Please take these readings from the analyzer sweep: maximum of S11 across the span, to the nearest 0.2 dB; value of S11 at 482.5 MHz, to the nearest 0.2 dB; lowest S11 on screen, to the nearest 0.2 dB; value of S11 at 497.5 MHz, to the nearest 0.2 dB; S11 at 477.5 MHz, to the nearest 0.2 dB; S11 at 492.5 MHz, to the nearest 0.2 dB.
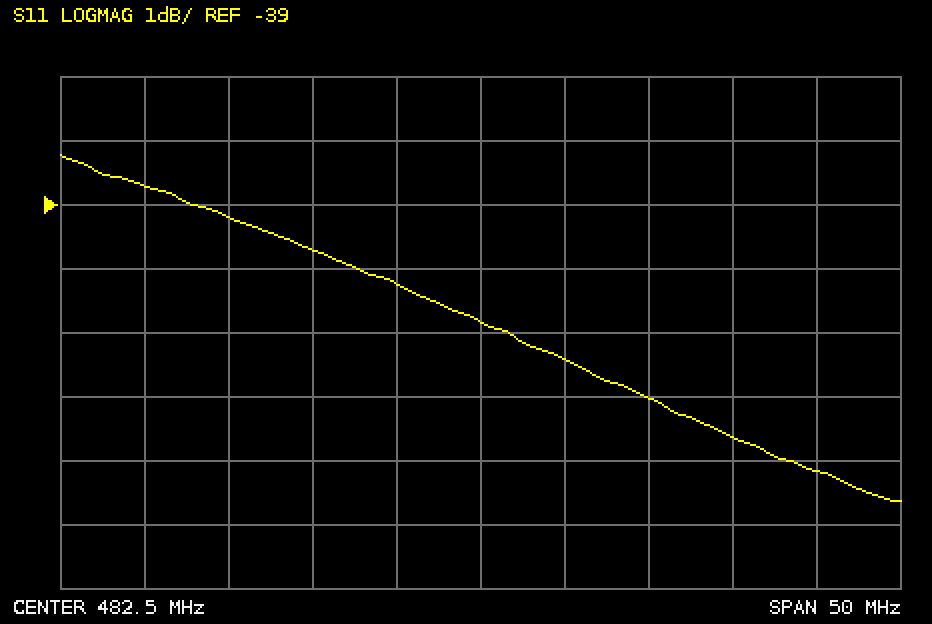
-38.2 dB
-40.8 dB
-43.6 dB
-42.6 dB
-40.2 dB
-42.0 dB
